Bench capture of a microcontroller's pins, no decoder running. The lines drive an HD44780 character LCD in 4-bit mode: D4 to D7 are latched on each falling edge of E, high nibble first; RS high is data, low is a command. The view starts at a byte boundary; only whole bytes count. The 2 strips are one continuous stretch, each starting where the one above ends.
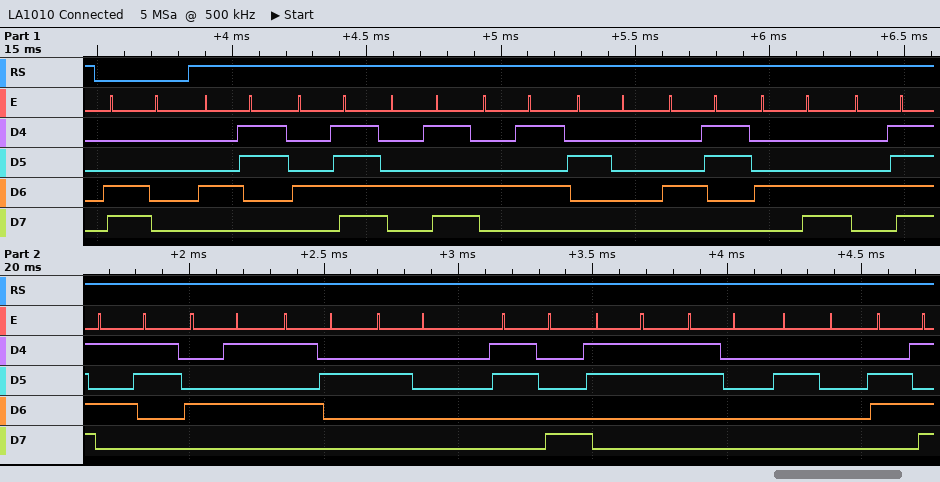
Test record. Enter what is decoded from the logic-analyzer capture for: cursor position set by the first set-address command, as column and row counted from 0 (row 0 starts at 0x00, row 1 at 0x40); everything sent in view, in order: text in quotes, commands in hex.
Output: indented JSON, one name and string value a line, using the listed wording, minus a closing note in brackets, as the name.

{
  "cursor position set by the first set-address command, as column and row counted from 0": "column 0, row 1",
  "everything sent in view, in order: text in quotes, commands in hex": "0xC0 \"COME CLOSER 830 m\""
}
